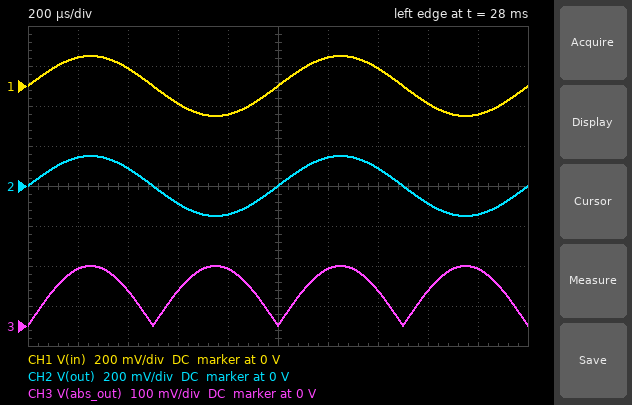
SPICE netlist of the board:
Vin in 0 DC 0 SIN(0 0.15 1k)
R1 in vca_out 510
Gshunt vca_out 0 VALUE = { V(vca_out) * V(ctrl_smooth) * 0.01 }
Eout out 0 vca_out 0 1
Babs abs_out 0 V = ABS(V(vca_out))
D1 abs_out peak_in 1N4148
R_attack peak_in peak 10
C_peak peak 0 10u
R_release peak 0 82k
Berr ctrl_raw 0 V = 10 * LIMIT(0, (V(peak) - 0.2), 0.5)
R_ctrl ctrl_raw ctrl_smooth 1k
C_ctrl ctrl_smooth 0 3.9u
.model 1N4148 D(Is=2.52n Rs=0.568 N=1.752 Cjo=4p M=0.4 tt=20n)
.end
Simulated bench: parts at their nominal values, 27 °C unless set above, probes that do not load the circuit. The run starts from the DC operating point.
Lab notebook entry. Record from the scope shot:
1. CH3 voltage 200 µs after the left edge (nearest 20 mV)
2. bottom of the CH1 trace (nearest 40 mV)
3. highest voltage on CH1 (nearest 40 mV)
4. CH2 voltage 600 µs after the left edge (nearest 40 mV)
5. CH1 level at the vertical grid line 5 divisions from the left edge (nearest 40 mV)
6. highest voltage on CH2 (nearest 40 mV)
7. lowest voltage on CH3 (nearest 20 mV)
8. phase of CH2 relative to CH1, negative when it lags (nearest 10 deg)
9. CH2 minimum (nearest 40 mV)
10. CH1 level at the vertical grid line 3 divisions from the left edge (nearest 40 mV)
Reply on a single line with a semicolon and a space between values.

140 mV; -160 mV; 160 mV; -80 mV; 0 V; 160 mV; 0 V; 0 deg; -160 mV; -80 mV
